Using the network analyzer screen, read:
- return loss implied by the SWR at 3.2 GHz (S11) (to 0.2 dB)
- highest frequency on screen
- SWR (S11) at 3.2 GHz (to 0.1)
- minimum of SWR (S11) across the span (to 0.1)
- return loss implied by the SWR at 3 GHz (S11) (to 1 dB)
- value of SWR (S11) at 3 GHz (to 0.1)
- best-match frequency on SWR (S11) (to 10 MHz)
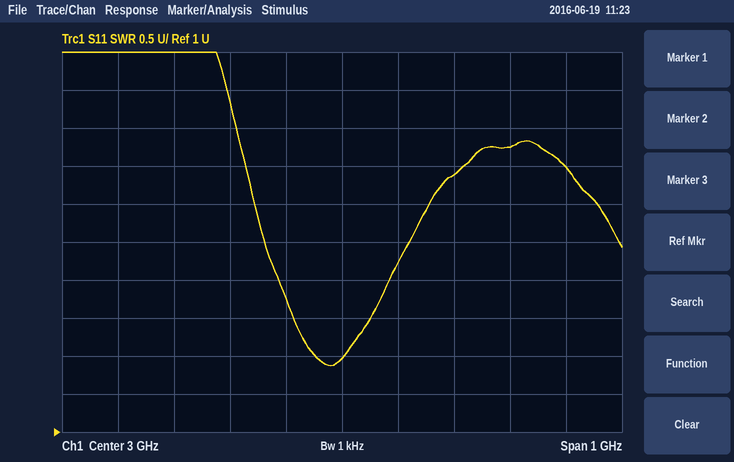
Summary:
4.0 dB
3.5 GHz
4.4
1.9
10 dB
2.0
2.98 GHz
